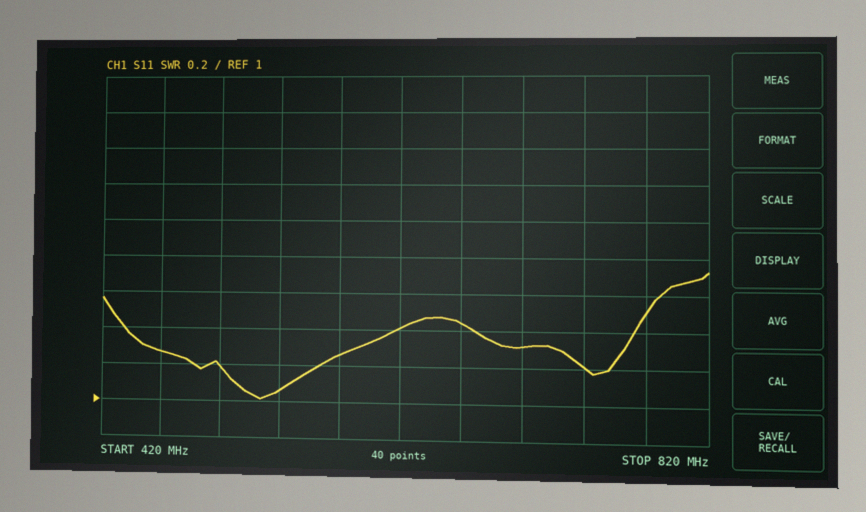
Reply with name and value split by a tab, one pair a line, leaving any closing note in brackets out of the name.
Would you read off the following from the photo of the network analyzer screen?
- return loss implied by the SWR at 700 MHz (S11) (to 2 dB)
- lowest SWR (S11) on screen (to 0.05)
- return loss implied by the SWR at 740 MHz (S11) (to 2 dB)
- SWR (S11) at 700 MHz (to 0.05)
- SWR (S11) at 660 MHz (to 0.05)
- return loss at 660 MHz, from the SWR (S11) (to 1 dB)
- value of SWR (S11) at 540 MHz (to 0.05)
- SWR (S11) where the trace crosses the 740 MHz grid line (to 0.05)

return loss implied by the SWR at 700 MHz (S11)	18 dB
lowest SWR (S11) on screen	1.00
return loss implied by the SWR at 740 MHz (S11)	20 dB
SWR (S11) at 700 MHz	1.30
SWR (S11) at 660 MHz	1.45
return loss at 660 MHz, from the SWR (S11)	15 dB
value of SWR (S11) at 540 MHz	1.05
SWR (S11) where the trace crosses the 740 MHz grid line	1.20
